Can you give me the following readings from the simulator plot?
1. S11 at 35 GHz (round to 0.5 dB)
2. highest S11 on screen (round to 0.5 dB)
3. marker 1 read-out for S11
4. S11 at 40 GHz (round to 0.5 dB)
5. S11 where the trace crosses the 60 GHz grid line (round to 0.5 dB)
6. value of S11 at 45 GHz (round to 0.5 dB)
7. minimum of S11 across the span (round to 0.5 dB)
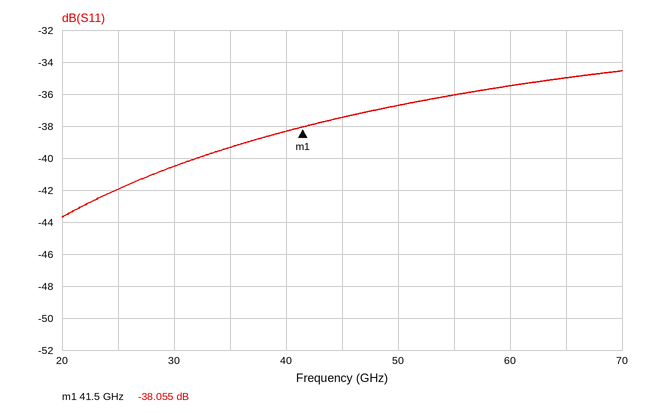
-39.5 dB
-34.5 dB
-38.055 dB
-38.5 dB
-35.5 dB
-37.5 dB
-43.5 dB
